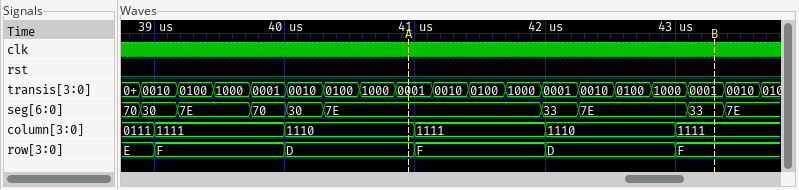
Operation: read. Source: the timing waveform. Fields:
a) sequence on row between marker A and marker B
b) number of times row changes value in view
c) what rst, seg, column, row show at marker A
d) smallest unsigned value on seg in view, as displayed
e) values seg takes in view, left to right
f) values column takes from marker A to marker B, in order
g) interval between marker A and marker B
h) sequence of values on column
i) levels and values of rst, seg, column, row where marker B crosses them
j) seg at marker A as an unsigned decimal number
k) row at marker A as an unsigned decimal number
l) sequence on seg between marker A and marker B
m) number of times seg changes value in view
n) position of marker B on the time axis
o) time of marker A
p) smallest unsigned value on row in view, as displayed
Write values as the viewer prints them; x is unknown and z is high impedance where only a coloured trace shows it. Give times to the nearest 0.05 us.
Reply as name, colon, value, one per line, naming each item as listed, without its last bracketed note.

sequence on row between marker A and marker B: D, F, D, F
number of times row changes value in view: 5
what rst, seg, column, row show at marker A: rst=0, seg=7E, column=1110, row=D
smallest unsigned value on seg in view, as displayed: 30
values seg takes in view, left to right: 70, 30, 7E, 70, 30, 7E, 33, 7E, 33, 7E
values column takes from marker A to marker B, in order: 1110, 1111, 1110, 1111
interval between marker A and marker B: 2.35 us
sequence of values on column: 0111, 1111, 1110, 1111, 1110, 1111
levels and values of rst, seg, column, row where marker B crosses them: rst=0, seg=33, column=1111, row=F
seg at marker A as an unsigned decimal number: 126
row at marker A as an unsigned decimal number: 13
sequence on seg between marker A and marker B: 7E, 33, 7E, 33
number of times seg changes value in view: 9
position of marker B on the time axis: 43.3 us
time of marker A: 40.95 us
smallest unsigned value on row in view, as displayed: D
